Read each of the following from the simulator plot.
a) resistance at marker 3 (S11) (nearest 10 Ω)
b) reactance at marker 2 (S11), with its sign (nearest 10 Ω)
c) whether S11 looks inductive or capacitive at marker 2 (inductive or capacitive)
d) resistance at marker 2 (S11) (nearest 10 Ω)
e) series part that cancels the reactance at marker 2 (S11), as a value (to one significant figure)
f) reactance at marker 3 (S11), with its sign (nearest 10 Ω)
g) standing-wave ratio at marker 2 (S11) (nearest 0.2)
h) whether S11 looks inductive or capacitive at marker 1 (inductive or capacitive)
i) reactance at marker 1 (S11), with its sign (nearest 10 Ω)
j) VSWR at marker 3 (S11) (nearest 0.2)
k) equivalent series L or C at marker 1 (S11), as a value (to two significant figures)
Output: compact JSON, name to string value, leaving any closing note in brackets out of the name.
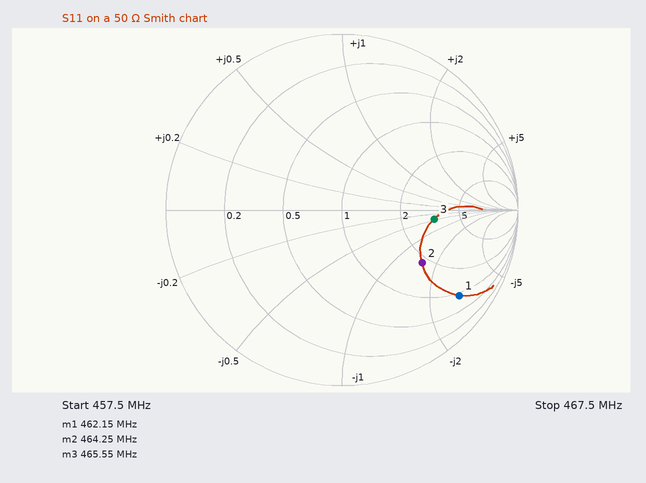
{"resistance at marker 3 (S11)": "160 Ω", "reactance at marker 2 (S11), with its sign": "-80 Ω", "whether S11 looks inductive or capacitive at marker 2": "capacitive", "resistance at marker 2 (S11)": "90 Ω", "series part that cancels the reactance at marker 2 (S11), as a value": "30 nH", "reactance at marker 3 (S11), with its sign": "-20 Ω", "standing-wave ratio at marker 2 (S11)": "3.4", "whether S11 looks inductive or capacitive at marker 1": "capacitive", "reactance at marker 1 (S11), with its sign": "-140 Ω", "VSWR at marker 3 (S11)": "3.2", "equivalent series L or C at marker 1 (S11), as a value": "2.5 pF"}
